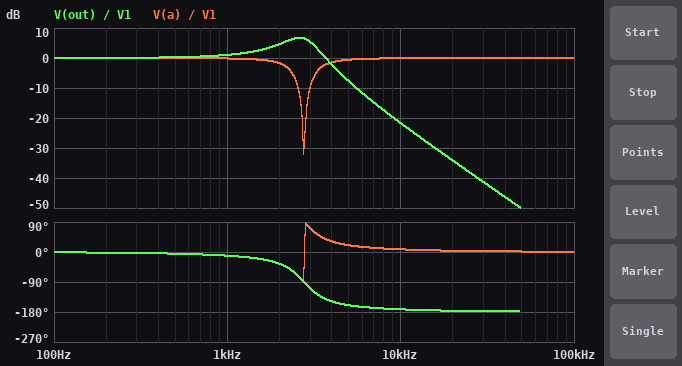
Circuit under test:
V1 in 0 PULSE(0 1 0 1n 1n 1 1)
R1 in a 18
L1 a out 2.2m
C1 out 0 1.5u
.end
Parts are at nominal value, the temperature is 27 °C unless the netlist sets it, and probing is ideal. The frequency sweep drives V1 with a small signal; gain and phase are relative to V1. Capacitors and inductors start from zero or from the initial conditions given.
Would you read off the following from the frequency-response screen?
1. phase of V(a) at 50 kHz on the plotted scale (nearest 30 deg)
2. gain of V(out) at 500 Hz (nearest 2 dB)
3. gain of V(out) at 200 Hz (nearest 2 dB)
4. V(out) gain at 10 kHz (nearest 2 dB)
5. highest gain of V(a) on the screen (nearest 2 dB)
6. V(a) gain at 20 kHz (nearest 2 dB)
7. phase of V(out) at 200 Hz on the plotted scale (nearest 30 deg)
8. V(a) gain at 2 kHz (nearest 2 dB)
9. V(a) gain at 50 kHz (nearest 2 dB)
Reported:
0 deg
0 dB
0 dB
-22 dB
0 dB
0 dB
0 deg
-2 dB
0 dB
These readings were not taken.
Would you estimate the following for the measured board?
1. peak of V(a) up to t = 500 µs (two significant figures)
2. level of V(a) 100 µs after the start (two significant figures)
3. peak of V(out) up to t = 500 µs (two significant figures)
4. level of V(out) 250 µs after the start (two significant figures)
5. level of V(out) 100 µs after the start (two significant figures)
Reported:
1.2 V
680 mV
1.5 V
1.2 V
920 mV
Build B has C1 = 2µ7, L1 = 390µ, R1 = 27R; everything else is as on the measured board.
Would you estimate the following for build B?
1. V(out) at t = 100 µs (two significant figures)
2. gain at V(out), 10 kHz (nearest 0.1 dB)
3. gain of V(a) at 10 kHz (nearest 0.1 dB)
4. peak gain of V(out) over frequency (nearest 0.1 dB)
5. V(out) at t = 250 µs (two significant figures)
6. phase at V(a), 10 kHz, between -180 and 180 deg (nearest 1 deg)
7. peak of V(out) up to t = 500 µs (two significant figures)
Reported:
760 mV
-14.9 dB
-4.9 dB
0 dB
990 mV
55 deg
1.0 V
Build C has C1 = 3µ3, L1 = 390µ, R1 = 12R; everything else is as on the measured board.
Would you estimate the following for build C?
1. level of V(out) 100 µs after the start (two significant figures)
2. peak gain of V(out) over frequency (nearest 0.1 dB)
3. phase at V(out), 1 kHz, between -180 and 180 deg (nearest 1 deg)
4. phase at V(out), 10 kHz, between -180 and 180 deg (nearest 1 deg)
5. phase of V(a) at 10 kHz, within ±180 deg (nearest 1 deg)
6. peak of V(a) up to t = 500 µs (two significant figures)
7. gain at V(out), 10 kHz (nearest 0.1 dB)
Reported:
1.0 V
0.7 dB
-15 deg
-149 deg
31 deg
1.1 V
-13.6 dB
